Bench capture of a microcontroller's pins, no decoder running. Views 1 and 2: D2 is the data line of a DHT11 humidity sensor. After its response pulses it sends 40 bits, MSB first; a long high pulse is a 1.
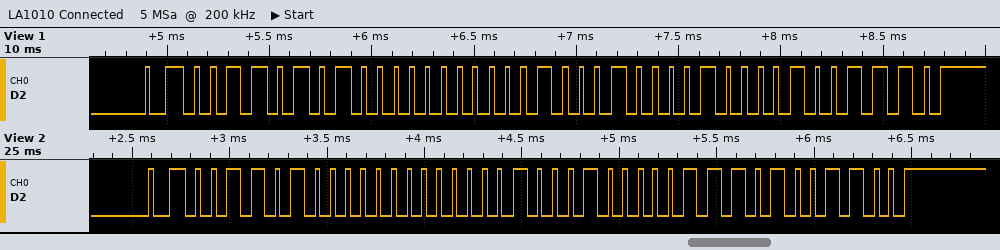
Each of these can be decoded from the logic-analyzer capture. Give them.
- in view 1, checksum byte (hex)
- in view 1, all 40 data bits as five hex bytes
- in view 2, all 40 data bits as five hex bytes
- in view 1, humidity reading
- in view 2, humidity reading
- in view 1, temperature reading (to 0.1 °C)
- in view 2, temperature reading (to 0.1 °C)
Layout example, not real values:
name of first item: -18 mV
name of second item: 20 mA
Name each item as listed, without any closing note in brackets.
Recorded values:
in view 1, checksum byte: 0x4E
in view 1, all 40 data bits as five hex bytes: 35 00 11 08 4E
in view 2, all 40 data bits as five hex bytes: 34 00 11 07 4C
in view 1, humidity reading: 53 %
in view 2, humidity reading: 52 %
in view 1, temperature reading: 17.8 °C
in view 2, temperature reading: 17.7 °C
